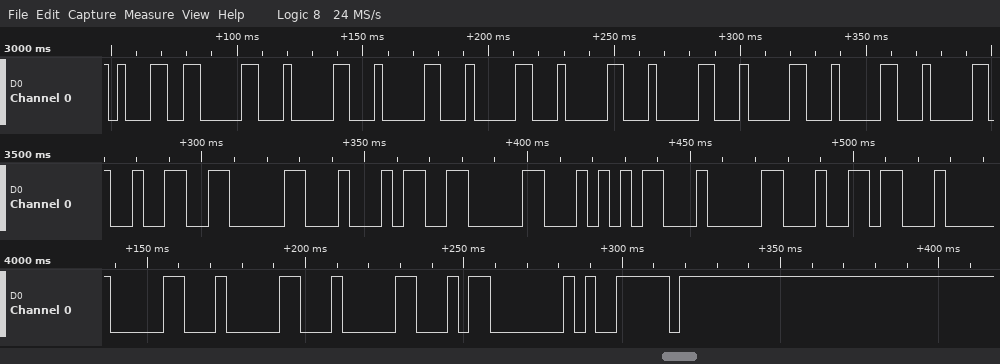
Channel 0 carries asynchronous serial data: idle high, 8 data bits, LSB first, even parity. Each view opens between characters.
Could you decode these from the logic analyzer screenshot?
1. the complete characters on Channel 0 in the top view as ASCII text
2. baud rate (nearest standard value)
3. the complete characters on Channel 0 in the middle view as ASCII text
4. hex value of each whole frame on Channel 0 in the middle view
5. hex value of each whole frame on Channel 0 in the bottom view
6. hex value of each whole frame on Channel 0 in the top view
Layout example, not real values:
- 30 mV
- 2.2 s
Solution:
- "100000000"
- 300 baud
- "2040506"
- 32, 30, 34, 30, 35, 30, 36
- 30, 30, 30, 03, F9
- 31, 30, 30, 30, 30, 30, 30, 30, 30
